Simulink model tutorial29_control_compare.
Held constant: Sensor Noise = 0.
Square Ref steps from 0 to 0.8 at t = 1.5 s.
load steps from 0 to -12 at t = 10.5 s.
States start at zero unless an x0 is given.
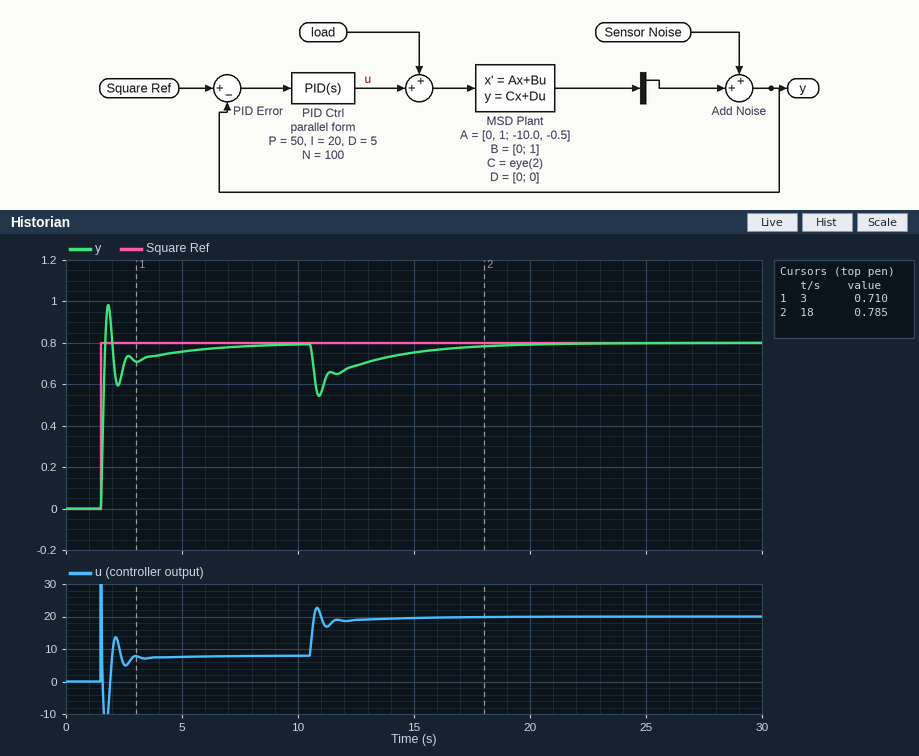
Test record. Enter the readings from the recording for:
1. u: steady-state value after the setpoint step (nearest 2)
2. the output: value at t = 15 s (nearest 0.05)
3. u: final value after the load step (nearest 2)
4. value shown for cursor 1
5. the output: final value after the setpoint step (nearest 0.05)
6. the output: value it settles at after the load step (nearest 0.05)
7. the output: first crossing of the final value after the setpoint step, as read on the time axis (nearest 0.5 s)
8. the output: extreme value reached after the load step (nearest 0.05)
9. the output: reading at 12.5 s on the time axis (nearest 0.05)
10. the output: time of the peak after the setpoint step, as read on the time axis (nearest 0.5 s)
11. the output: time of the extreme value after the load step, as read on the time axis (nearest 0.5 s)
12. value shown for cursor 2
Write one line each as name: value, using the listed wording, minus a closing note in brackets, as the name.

u: steady-state value after the setpoint step: 8
the output: value at t = 15 s: 0.75
u: final value after the load step: 20
value shown for cursor 1: 0.710
the output: final value after the setpoint step: 0.80
the output: value it settles at after the load step: 0.80
the output: first crossing of the final value after the setpoint step, as read on the time axis: 1.5 s
the output: extreme value reached after the load step: 0.55
the output: reading at 12.5 s on the time axis: 0.70
the output: time of the peak after the setpoint step, as read on the time axis: 2.0 s
the output: time of the extreme value after the load step, as read on the time axis: 11.0 s
value shown for cursor 2: 0.785
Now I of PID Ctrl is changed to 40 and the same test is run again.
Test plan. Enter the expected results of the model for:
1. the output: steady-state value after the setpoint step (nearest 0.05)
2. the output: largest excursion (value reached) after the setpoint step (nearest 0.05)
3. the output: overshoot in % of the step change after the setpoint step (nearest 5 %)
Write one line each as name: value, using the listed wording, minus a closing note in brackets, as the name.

the output: steady-state value after the setpoint step: 0.80
the output: largest excursion (value reached) after the setpoint step: 1.00
the output: overshoot in % of the step change after the setpoint step: 25 %
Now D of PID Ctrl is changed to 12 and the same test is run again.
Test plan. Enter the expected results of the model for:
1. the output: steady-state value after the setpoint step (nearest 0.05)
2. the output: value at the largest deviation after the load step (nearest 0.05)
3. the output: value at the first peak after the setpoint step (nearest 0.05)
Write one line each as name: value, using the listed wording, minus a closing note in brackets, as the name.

the output: steady-state value after the setpoint step: 0.80
the output: value at the largest deviation after the load step: 0.60
the output: value at the first peak after the setpoint step: 0.85
